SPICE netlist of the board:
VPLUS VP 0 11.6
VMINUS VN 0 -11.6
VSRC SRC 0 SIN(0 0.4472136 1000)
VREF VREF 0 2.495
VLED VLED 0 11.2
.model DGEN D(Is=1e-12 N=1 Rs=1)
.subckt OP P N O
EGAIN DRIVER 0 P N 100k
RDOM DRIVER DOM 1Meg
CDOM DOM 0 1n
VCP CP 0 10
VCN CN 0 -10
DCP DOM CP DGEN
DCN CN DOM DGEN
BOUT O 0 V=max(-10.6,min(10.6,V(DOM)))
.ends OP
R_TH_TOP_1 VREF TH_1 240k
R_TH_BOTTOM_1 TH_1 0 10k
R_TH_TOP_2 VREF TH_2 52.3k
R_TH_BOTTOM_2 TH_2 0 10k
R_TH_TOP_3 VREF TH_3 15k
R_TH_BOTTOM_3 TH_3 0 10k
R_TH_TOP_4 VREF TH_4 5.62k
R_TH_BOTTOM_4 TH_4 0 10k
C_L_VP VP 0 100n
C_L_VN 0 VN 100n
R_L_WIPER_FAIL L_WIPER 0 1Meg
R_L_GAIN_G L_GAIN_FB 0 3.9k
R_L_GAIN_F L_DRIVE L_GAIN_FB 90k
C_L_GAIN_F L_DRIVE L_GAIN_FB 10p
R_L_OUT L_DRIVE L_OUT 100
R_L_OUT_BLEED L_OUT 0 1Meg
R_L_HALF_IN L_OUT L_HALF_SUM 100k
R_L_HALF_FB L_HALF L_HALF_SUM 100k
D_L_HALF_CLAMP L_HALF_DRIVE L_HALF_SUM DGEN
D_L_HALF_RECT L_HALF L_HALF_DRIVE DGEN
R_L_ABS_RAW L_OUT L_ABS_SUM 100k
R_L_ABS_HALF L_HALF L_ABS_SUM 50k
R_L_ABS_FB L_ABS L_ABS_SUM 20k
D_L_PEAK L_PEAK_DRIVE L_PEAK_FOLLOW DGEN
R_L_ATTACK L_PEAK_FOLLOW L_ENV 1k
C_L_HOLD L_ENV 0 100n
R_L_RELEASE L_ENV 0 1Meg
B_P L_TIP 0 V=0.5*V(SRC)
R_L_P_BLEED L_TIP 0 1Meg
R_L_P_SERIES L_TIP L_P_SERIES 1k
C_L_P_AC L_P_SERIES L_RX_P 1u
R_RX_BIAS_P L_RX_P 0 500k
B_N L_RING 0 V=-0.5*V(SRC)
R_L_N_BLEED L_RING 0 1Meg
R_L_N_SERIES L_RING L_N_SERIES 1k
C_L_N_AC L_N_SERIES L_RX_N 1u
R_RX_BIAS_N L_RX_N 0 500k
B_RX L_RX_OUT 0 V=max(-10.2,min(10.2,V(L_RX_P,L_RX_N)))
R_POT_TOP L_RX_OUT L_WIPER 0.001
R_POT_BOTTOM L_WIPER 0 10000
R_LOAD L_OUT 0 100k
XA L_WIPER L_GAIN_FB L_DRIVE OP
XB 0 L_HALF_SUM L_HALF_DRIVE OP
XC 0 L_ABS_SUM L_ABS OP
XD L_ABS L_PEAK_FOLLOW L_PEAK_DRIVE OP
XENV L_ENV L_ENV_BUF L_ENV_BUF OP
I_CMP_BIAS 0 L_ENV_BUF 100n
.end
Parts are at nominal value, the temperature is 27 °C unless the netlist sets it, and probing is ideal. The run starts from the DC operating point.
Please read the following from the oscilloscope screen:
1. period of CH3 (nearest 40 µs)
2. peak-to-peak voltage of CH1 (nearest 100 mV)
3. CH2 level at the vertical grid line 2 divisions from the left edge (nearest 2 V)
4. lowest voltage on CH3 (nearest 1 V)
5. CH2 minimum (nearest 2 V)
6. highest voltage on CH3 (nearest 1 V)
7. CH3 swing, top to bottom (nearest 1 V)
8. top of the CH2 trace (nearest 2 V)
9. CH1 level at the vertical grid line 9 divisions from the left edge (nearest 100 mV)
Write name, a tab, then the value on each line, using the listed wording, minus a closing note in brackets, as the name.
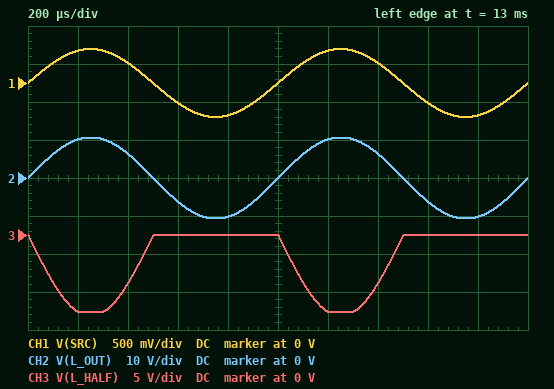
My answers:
period of CH3	1.00 ms
peak-to-peak voltage of CH1	900 mV
CH2 level at the vertical grid line 2 divisions from the left edge	6 V
lowest voltage on CH3	-10 V
CH2 minimum	-10 V
highest voltage on CH3	0 V
CH3 swing, top to bottom	10 V
top of the CH2 trace	10 V
CH1 level at the vertical grid line 9 divisions from the left edge	-400 mV
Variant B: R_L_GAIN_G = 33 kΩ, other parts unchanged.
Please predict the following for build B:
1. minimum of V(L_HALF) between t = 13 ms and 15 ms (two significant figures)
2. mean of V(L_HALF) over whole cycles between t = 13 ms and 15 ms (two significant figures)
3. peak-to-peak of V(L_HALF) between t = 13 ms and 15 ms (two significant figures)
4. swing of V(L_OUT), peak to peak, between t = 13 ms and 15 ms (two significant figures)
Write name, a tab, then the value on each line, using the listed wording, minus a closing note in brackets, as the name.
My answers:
minimum of V(L_HALF) between t = 13 ms and 15 ms	-1.7 V
mean of V(L_HALF) over whole cycles between t = 13 ms and 15 ms	-530 mV
peak-to-peak of V(L_HALF) between t = 13 ms and 15 ms	1.7 V
swing of V(L_OUT), peak to peak, between t = 13 ms and 15 ms	3.3 V
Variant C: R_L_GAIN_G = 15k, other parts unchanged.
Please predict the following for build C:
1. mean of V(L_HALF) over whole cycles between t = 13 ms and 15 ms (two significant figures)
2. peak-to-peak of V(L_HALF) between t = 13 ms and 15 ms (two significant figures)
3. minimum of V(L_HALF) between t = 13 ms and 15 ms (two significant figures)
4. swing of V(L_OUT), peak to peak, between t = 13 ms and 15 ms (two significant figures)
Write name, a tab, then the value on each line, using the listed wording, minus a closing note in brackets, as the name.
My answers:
mean of V(L_HALF) over whole cycles between t = 13 ms and 15 ms	-990 mV
peak-to-peak of V(L_HALF) between t = 13 ms and 15 ms	3.1 V
minimum of V(L_HALF) between t = 13 ms and 15 ms	-3.1 V
swing of V(L_OUT), peak to peak, between t = 13 ms and 15 ms	6.2 V
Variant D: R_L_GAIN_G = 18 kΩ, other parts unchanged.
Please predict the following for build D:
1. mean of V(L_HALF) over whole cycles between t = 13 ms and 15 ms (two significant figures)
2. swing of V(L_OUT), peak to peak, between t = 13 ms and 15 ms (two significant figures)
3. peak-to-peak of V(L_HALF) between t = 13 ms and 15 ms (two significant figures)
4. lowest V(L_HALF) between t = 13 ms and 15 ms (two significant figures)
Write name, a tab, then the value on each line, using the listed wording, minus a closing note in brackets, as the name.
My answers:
mean of V(L_HALF) over whole cycles between t = 13 ms and 15 ms	-850 mV
swing of V(L_OUT), peak to peak, between t = 13 ms and 15 ms	5.3 V
peak-to-peak of V(L_HALF) between t = 13 ms and 15 ms	2.7 V
lowest V(L_HALF) between t = 13 ms and 15 ms	-2.7 V
